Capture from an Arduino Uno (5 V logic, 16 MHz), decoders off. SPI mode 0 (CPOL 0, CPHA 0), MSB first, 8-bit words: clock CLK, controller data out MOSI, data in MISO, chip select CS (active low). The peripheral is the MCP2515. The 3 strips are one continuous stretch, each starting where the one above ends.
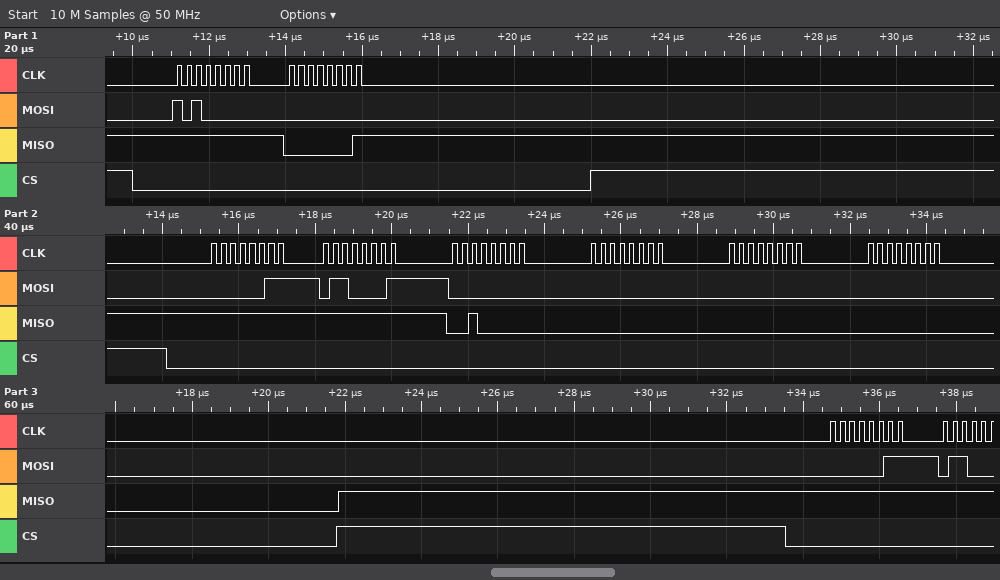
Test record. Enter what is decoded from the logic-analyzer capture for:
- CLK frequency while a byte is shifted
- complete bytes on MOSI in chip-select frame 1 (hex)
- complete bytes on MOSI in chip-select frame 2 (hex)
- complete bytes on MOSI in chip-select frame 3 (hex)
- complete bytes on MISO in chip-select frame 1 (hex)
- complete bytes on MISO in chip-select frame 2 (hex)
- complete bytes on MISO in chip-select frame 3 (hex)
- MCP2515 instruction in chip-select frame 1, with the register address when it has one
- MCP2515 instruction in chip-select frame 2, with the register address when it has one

4 MHz
A0 00
03 61 00 00 00 00
03
FF 01
FF FF 20 00 00 00
FF
READ STATUS
READ 0x61
